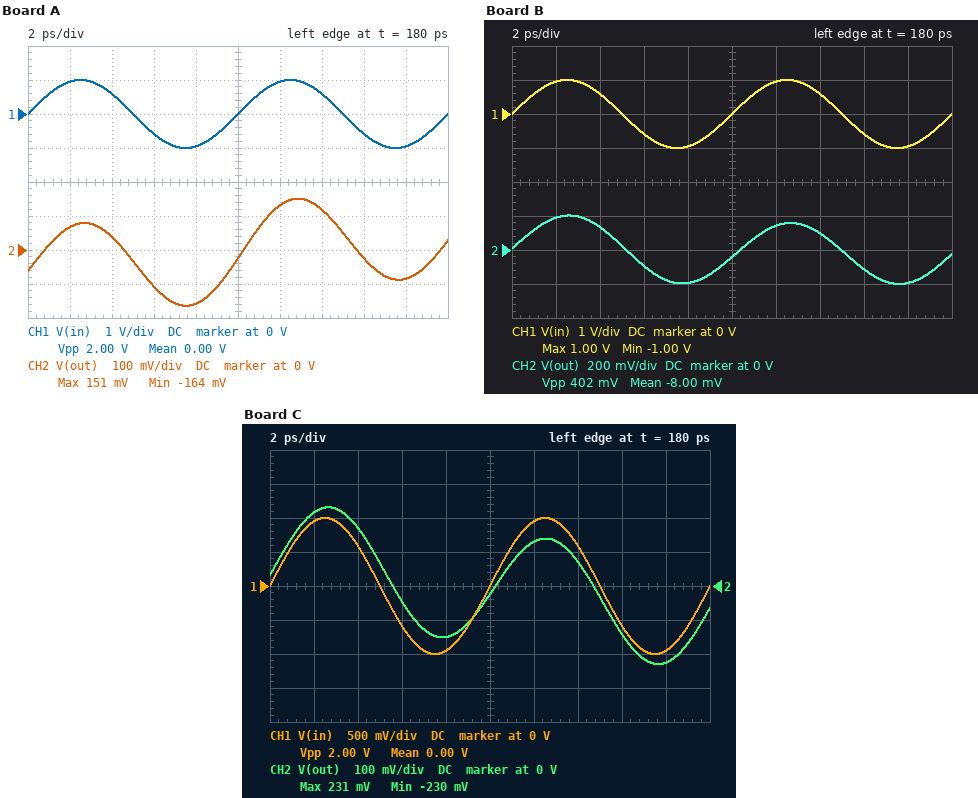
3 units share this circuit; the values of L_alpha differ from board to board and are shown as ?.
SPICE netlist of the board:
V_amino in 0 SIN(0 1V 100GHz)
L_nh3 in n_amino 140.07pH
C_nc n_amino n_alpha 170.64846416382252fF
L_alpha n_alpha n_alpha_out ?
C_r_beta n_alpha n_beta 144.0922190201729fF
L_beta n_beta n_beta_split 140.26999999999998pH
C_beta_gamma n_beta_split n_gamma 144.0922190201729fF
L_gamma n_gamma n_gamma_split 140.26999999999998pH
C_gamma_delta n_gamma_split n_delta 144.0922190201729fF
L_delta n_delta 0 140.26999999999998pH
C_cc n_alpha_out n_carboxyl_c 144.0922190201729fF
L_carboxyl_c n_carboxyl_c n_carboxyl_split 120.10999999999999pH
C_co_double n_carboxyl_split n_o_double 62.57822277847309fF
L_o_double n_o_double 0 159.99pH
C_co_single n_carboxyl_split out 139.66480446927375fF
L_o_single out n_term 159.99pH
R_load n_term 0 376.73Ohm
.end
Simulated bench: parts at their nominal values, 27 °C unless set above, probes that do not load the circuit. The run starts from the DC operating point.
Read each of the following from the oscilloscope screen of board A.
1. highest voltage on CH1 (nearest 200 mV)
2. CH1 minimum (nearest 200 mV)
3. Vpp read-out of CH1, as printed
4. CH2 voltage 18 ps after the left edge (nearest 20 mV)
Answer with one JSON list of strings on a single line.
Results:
["1.0 V", "-1.0 V", "2.00 V", "-80 mV"]
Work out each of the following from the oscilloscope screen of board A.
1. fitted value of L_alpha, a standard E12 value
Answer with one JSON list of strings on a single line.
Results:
["330 pH"]
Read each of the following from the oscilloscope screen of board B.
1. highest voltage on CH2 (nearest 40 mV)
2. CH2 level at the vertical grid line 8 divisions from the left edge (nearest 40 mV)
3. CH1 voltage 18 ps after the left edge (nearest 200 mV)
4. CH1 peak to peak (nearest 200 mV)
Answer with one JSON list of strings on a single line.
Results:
["200 mV", "-120 mV", "-1.0 V", "2.0 V"]
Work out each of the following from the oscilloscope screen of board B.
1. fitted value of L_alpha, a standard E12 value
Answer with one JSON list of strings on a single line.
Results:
["150 pH"]
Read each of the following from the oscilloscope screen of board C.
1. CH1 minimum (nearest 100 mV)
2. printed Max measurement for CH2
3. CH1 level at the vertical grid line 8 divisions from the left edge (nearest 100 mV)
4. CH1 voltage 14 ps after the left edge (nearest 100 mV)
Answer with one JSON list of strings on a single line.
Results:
["-1.0 V", "231 mV", "-600 mV", "600 mV"]
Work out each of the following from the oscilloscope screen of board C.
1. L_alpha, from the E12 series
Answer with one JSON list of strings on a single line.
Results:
["180 pH"]
